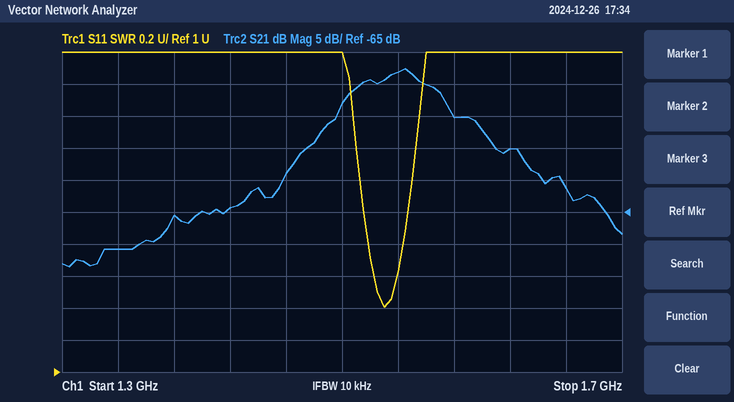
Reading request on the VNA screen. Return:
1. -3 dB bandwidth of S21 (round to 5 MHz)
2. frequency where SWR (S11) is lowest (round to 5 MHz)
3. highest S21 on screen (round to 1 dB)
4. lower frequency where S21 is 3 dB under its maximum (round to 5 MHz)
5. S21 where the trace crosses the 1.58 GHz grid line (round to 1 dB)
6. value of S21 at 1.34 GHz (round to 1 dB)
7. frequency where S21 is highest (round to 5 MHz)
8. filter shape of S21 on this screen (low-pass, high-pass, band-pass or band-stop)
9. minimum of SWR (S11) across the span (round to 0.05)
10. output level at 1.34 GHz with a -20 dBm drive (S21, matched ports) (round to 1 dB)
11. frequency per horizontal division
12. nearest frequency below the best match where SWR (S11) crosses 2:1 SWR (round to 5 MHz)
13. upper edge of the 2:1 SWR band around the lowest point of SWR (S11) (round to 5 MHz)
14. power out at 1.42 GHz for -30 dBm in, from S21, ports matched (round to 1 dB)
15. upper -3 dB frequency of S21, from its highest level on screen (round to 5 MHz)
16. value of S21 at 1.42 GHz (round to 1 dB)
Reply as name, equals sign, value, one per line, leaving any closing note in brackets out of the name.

-3 dB bandwidth of S21 = 55 MHz
frequency where SWR (S11) is lowest = 1.530 GHz
highest S21 on screen = -43 dB
lower frequency where S21 is 3 dB under its maximum = 1.510 GHz
S21 where the trace crosses the 1.58 GHz grid line = -50 dB
value of S21 at 1.34 GHz = -71 dB
frequency where S21 is highest = 1.545 GHz
filter shape of S21 on this screen = band-pass
minimum of SWR (S11) across the span = 1.40
output level at 1.34 GHz with a -20 dBm drive (S21, matched ports) = -91 dBm
frequency per horizontal division = 40 MHz
nearest frequency below the best match where SWR (S11) crosses 2:1 SWR = 1.515 GHz
upper edge of the 2:1 SWR band around the lowest point of SWR (S11) = 1.545 GHz
power out at 1.42 GHz for -30 dBm in, from S21, ports matched = -94 dBm
upper -3 dB frequency of S21, from its highest level on screen = 1.565 GHz
value of S21 at 1.42 GHz = -64 dB
